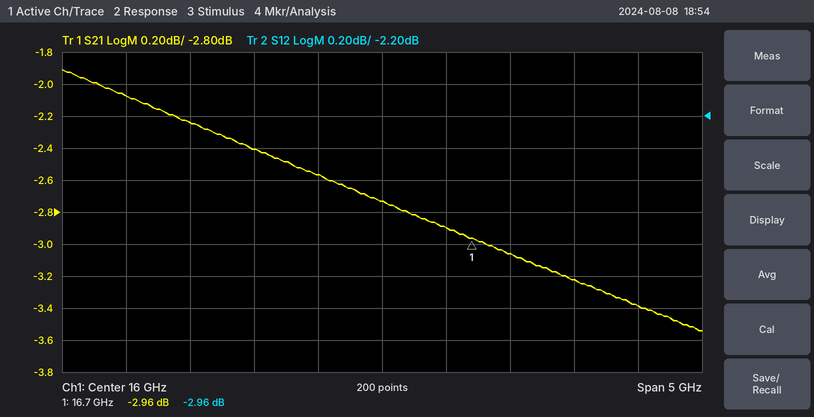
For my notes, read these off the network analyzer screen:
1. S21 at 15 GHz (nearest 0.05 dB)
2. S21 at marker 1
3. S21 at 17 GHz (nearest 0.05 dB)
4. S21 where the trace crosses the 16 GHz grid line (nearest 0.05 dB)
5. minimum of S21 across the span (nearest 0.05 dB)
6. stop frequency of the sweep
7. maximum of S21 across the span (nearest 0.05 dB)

-2.40 dB
-2.96 dB
-3.05 dB
-2.75 dB
-3.55 dB
18.5 GHz
-1.90 dB
